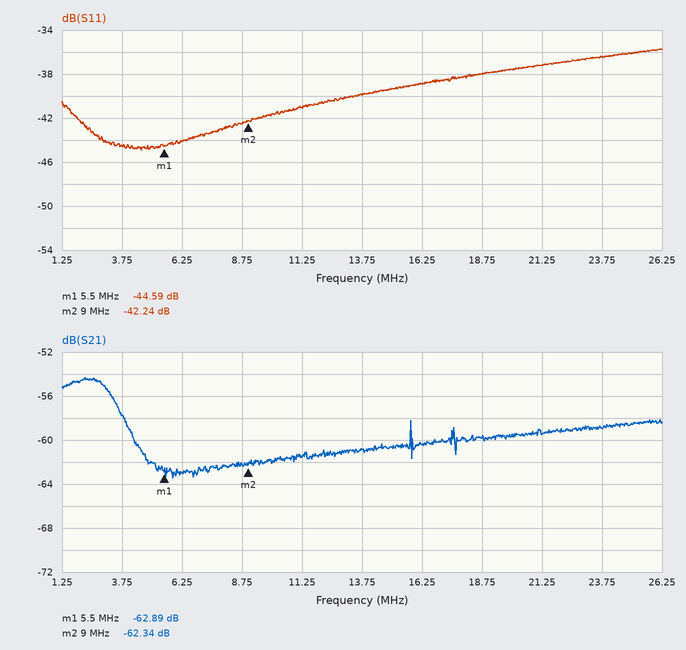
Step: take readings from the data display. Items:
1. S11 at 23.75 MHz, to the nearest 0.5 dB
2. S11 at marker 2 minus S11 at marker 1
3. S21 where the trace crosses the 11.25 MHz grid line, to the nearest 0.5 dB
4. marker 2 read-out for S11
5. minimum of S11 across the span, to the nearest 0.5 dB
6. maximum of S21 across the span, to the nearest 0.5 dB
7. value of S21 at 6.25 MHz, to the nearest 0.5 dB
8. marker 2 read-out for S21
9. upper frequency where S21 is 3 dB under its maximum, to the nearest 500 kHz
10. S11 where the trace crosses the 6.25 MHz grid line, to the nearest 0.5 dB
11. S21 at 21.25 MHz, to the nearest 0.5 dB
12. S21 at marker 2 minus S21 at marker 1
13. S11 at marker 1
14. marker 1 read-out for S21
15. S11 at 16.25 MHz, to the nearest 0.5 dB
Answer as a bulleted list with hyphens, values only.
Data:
- -36.5 dB
- 2.35 dB
- -61.5 dB
- -42.24 dB
- -45.0 dB
- -54.5 dB
- -63.0 dB
- -62.34 dB
- 3.5 MHz
- -44.0 dB
- -59.5 dB
- 0.55 dB
- -44.59 dB
- -62.89 dB
- -39.0 dB
